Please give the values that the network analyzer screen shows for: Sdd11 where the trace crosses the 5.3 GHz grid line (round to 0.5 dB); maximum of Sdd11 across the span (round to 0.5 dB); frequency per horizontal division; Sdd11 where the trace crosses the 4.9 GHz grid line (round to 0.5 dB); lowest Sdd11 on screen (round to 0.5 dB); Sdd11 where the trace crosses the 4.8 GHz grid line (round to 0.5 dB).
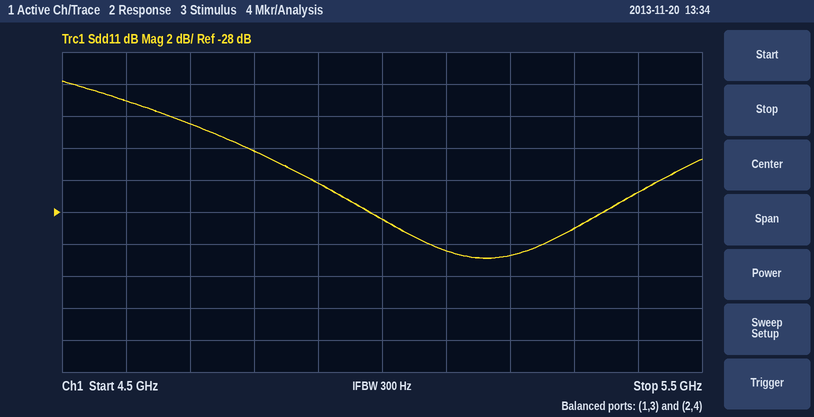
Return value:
-29.0 dB
-20.0 dB
100 MHz
-26.0 dB
-31.0 dB
-24.0 dB
